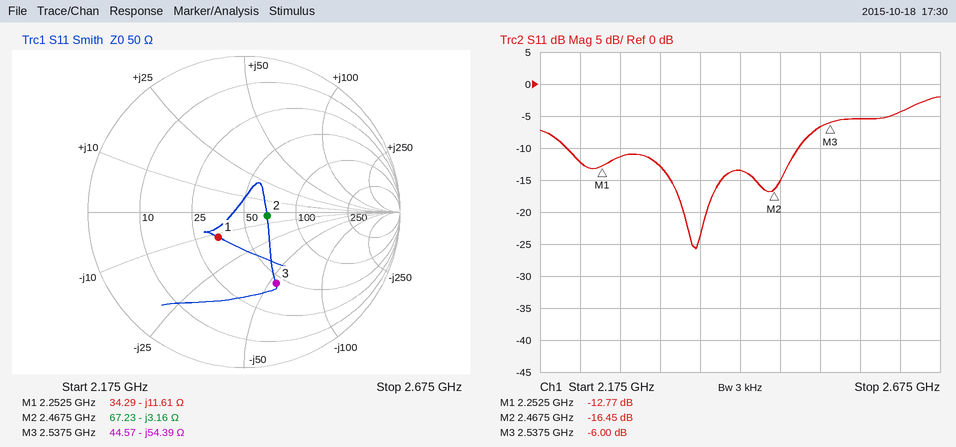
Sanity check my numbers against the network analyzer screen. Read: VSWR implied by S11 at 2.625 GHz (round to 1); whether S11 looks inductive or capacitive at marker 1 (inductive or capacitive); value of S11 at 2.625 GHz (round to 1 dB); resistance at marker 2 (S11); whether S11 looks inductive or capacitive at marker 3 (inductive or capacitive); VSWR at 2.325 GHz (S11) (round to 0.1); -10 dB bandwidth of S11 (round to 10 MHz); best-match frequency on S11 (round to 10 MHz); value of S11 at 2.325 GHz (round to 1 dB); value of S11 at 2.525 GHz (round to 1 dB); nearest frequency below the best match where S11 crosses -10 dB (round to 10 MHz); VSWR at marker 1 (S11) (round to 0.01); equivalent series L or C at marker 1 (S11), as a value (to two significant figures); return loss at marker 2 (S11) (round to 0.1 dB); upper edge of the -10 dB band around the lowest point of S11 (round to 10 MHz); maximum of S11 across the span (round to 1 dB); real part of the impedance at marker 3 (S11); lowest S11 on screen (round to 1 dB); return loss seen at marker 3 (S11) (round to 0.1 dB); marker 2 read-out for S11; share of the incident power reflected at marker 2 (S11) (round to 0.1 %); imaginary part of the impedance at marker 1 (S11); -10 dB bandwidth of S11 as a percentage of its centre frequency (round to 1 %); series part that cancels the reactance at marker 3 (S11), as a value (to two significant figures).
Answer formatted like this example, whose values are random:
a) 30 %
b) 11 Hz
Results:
a) 4
b) capacitive
c) -4 dB
d) 67.23 Ω
e) capacitive
f) 1.6
g) 290 MHz
h) 2.37 GHz
i) -13 dB
j) -7 dB
k) 2.21 GHz
l) 1.60
m) 6.1 pF
n) 16.5 dB
o) 2.50 GHz
p) -2 dB
q) 44.57 Ω
r) -26 dB
s) 6.0 dB
t) -16.45 dB
u) 2.3 %
v) -11.61 Ω
w) 12 %
x) 3.4 nH
